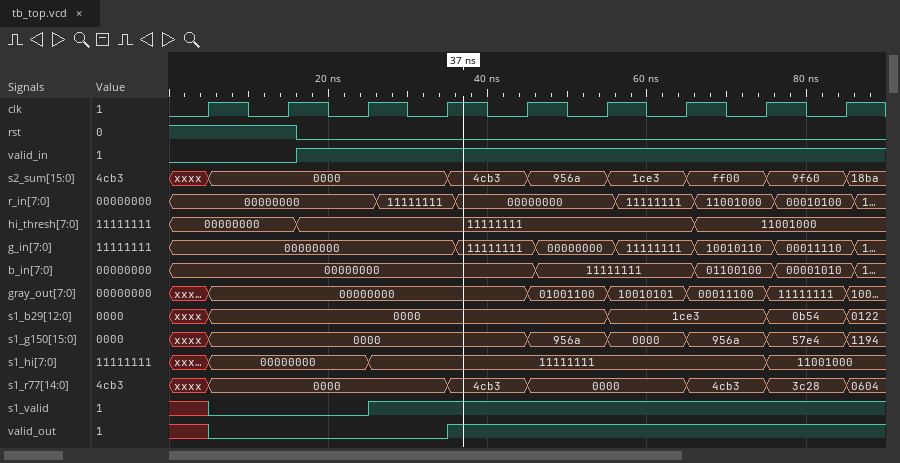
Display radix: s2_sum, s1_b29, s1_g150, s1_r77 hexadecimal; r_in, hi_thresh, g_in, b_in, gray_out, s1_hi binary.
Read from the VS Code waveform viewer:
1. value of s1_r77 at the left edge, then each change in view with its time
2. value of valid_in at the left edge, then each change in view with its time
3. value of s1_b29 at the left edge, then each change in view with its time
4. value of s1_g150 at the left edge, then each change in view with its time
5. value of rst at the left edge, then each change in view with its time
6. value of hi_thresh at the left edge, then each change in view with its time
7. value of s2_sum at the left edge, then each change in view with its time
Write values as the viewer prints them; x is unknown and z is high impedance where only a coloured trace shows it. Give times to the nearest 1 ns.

xxxx, 0000 at 5 ns, 4cb3 at 35 ns, 0000 at 45 ns, 4cb3 at 65 ns, 3c28 at 75 ns, 0604 at 85 ns
0, 1 at 16 ns
xxxx, 0000 at 5 ns, 1ce3 at 55 ns, 0b54 at 75 ns, 0122 at 85 ns
xxxx, 0000 at 5 ns, 956a at 45 ns, 0000 at 55 ns, 956a at 65 ns, 57e4 at 75 ns, 1194 at 85 ns
1, 0 at 16 ns
00000000, 11111111 at 16 ns, 11001000 at 66 ns
xxxx, 0000 at 5 ns, 4cb3 at 35 ns, 956a at 45 ns, 1ce3 at 55 ns, ff00 at 65 ns, 9f60 at 75 ns, 18ba at 85 ns
